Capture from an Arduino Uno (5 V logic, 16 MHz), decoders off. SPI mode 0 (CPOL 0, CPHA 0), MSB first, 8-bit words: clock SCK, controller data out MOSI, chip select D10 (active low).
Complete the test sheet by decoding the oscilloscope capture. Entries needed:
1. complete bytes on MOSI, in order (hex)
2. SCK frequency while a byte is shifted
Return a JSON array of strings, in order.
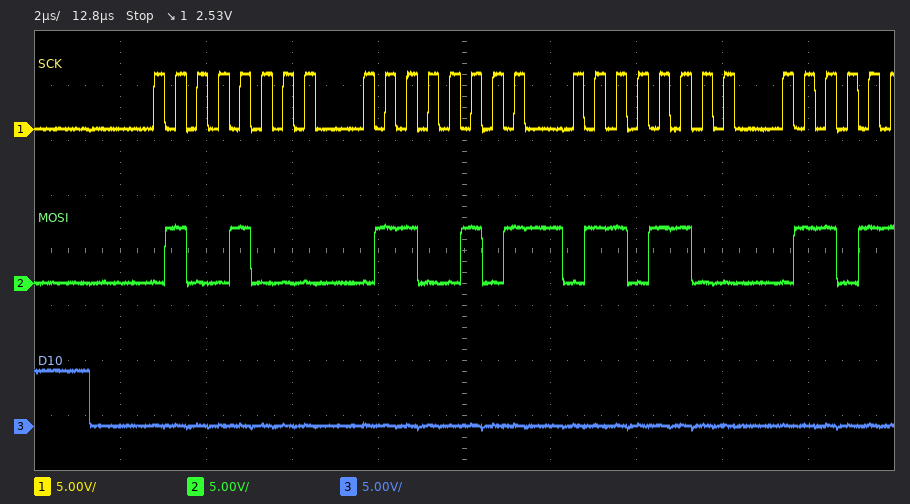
["48 65 6C", "2 MHz"]
